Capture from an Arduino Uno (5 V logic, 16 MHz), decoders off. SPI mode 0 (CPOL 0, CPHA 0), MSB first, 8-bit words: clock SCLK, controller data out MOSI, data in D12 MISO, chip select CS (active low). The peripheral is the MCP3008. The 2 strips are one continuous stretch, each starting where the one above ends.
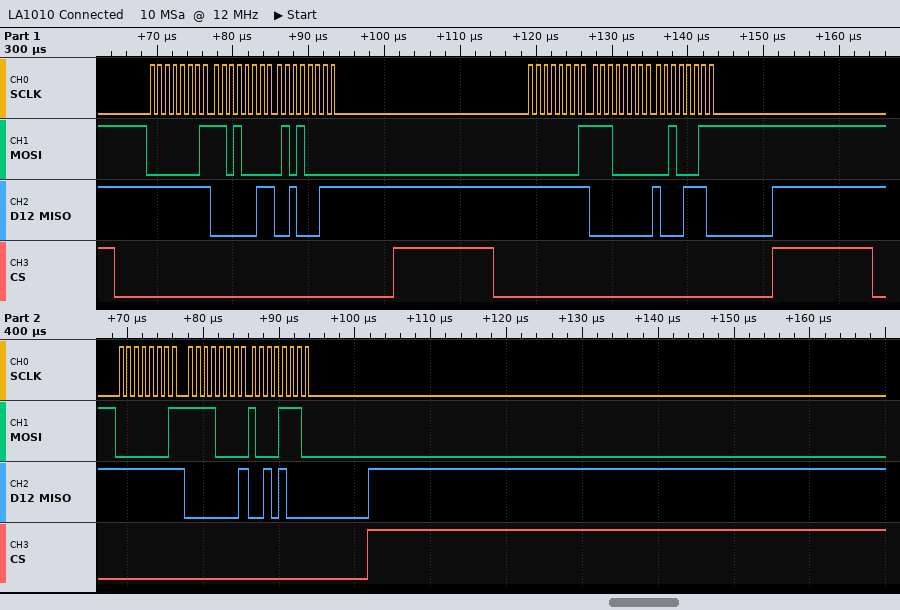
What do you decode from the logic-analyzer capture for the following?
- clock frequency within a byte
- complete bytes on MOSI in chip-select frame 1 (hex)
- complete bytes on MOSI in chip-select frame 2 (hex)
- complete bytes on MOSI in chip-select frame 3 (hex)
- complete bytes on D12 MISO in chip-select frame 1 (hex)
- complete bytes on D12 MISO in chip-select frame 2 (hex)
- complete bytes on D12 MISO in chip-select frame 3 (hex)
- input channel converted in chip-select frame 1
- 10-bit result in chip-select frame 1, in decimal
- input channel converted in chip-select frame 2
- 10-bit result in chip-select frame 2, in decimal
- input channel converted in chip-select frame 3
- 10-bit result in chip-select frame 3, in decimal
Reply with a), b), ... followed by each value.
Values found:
a) 1 MHz
b) 0x01 0xD0 0x50
c) 0x01 0xE0 0x23
d) 0x01 0xF0 0x8E
e) 0xFF 0x03 0x23
f) 0xFF 0x00 0x8E
g) 0xFF 0x01 0x28
h) 5
i) 803
j) 6
k) 142
l) 7
m) 296
